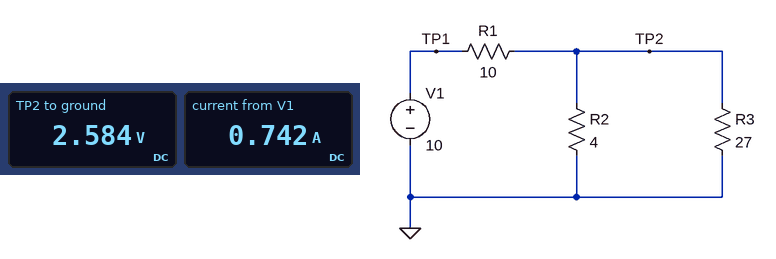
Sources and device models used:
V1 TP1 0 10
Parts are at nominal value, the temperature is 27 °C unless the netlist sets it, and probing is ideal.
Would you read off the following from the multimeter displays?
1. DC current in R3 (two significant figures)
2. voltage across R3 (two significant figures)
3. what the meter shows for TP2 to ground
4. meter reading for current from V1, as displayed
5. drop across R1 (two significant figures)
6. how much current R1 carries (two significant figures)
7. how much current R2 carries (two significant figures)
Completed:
96 mA
2.6 V
2.584 V
0.742 A
7.4 V
740 mA
650 mA
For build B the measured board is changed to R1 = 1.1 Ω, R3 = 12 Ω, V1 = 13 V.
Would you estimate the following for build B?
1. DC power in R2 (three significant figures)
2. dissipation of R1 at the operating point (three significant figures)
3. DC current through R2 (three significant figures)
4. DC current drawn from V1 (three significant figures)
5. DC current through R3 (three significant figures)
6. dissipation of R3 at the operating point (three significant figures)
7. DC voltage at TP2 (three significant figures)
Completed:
22.6 W
11.1 W
2.38 A
3.17 A
793 mA
7.54 W
9.51 V
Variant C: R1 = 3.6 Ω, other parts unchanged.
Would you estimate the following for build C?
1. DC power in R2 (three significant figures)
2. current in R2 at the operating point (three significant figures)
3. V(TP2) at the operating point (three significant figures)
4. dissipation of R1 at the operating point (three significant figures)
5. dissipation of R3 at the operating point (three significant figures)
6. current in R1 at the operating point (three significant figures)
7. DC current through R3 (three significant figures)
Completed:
6.05 W
1.23 A
4.92 V
7.17 W
896 mW
1.41 A
182 mA
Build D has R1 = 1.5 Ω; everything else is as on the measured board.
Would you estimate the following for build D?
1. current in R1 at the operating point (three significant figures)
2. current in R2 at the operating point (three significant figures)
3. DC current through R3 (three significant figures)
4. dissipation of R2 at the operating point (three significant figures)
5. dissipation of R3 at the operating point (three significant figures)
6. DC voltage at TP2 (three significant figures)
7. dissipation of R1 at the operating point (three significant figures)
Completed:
2.01 A
1.75 A
259 mA
12.2 W
1.81 W
6.99 V
6.04 W
